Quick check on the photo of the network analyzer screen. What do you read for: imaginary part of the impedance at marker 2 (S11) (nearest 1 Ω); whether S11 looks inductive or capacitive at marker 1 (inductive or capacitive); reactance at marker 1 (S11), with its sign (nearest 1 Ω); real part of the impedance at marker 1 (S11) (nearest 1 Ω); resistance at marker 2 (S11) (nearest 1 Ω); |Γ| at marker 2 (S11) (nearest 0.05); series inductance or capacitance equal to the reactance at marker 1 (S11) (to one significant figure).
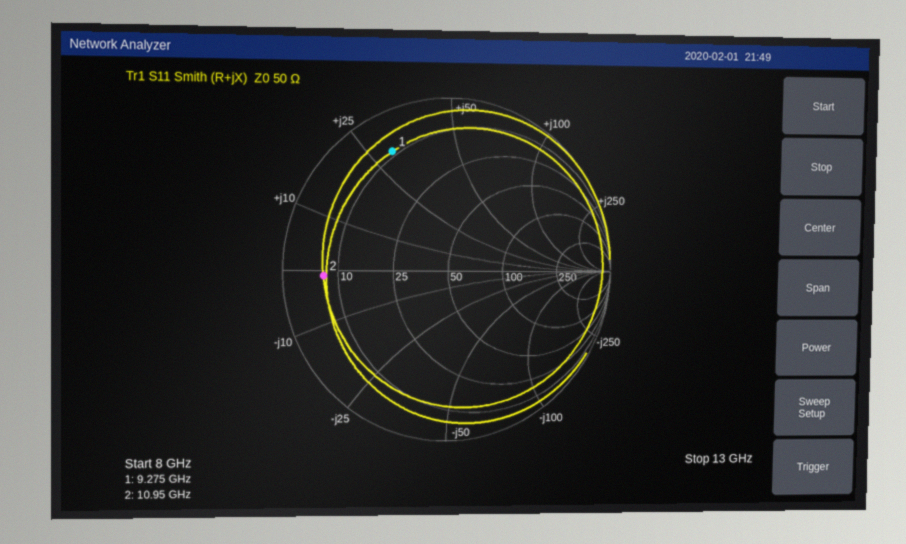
-1 Ω
inductive
+30 Ω
9 Ω
7 Ω
0.75
500 pH
